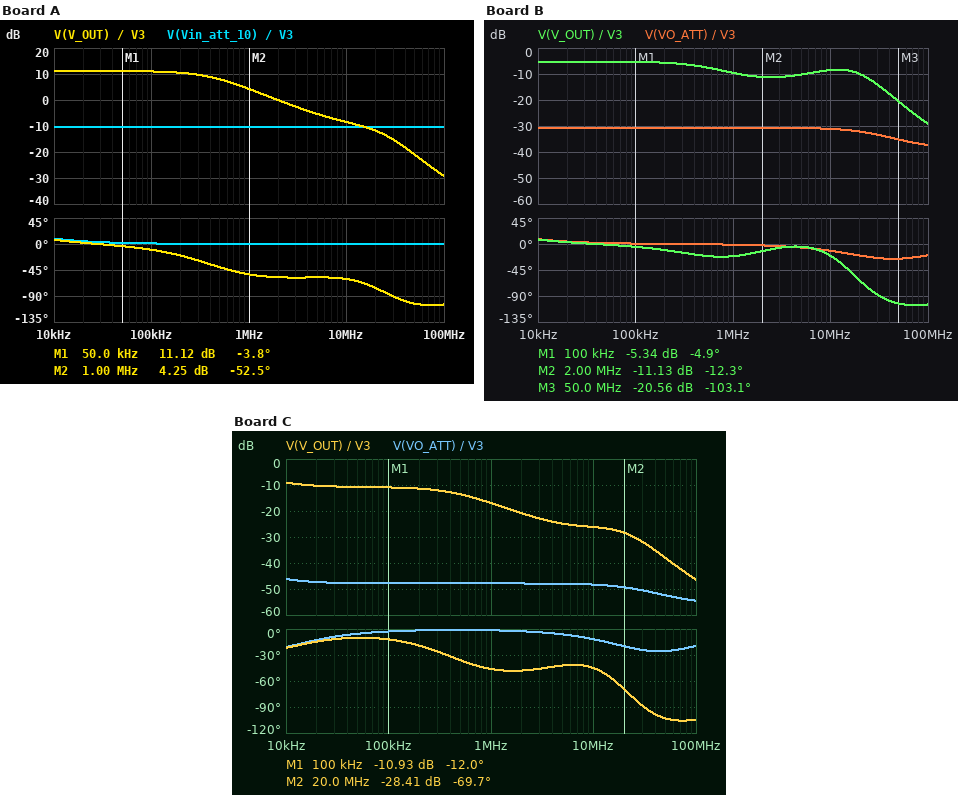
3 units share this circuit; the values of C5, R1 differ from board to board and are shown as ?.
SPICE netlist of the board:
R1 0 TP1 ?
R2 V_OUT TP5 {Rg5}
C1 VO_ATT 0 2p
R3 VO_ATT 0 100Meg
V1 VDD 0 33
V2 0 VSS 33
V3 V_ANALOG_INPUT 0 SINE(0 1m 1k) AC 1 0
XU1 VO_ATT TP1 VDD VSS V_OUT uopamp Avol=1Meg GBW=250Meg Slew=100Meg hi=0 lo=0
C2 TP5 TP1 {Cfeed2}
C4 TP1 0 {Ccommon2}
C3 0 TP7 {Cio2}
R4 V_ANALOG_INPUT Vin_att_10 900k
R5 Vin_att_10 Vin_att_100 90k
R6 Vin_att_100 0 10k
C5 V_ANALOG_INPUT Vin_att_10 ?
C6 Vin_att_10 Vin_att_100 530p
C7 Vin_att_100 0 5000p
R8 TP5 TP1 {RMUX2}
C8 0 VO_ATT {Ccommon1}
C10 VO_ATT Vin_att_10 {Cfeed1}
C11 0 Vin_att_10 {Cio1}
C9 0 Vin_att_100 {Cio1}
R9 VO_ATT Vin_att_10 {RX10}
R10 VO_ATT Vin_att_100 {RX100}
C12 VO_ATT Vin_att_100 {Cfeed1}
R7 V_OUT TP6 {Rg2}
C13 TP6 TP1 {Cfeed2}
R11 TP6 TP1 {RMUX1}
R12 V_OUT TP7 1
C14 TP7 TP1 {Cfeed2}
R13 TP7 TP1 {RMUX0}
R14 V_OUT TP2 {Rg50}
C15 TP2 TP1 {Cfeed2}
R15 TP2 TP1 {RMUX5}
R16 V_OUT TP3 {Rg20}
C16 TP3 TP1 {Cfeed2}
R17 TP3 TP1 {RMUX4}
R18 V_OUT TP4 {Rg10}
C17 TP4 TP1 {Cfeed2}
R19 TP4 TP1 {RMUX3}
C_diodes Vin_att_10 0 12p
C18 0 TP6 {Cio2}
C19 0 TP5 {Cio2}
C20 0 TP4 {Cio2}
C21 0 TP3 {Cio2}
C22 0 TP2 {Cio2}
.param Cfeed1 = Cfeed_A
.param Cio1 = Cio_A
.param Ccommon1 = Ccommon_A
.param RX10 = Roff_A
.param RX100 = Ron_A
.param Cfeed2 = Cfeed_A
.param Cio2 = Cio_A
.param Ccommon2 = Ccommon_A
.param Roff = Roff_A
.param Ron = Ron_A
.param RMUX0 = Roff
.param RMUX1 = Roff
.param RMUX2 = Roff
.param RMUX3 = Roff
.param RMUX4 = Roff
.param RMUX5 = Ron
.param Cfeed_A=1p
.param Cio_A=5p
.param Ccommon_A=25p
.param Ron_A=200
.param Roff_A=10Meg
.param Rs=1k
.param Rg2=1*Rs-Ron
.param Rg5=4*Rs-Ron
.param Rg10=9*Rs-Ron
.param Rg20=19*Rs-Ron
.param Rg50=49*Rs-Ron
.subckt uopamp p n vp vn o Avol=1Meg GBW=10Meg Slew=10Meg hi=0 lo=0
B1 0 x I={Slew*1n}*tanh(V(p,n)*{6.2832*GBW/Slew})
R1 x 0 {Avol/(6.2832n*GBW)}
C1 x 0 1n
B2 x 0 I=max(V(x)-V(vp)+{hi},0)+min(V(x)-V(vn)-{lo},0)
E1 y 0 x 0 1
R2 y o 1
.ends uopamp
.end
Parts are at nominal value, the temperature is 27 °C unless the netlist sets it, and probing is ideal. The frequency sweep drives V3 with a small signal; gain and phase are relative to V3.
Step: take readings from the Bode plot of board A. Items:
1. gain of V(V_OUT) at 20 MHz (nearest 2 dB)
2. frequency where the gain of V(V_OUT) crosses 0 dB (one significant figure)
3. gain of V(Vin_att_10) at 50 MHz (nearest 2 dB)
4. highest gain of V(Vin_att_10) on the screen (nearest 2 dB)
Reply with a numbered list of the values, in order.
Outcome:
1. -12 dB
2. 2 MHz
3. -10 dB
4. -10 dB
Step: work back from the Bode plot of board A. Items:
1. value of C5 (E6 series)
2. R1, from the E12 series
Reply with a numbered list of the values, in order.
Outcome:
1. 220 pF
2. 390 Ω
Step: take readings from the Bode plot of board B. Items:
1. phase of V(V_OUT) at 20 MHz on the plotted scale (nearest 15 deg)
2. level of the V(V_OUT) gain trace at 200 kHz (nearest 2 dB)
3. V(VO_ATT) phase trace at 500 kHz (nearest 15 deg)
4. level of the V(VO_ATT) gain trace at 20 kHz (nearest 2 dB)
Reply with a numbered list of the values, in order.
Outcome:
1. -60 deg
2. -6 dB
3. 0 deg
4. -30 dB
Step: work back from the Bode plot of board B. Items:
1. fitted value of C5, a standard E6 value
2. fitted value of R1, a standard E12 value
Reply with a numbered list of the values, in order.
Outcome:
1. 220 pF
2. 2.7 kΩ
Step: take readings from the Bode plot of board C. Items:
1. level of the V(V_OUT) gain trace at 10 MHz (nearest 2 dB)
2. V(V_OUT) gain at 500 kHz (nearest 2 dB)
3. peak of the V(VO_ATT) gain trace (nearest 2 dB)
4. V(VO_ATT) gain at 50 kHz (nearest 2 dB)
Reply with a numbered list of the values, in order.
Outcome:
1. -26 dB
2. -14 dB
3. -46 dB
4. -48 dB
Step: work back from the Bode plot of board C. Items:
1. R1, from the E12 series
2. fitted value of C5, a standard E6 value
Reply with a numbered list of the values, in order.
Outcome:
1. 680 Ω
2. 22 pF
